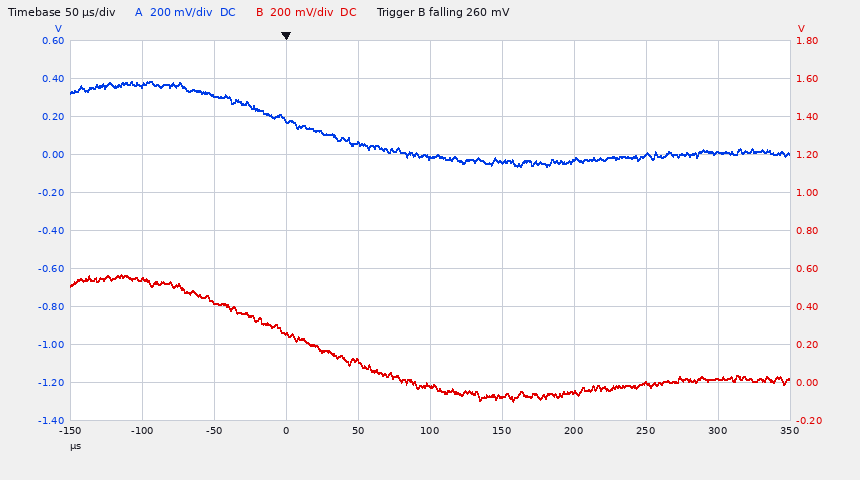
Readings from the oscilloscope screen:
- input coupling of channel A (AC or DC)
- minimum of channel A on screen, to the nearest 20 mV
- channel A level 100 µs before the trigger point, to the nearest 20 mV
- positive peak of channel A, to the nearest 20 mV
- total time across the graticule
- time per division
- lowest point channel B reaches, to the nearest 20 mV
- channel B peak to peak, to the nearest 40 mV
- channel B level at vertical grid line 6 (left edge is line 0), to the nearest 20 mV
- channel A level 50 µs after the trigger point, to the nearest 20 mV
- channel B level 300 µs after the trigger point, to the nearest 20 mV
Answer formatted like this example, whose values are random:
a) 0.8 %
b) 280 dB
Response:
a) DC
b) -60 mV
c) 360 mV
d) 380 mV
e) 500 µs
f) 50 µs
g) -100 mV
h) 680 mV
i) -80 mV
j) 60 mV
k) 20 mV
